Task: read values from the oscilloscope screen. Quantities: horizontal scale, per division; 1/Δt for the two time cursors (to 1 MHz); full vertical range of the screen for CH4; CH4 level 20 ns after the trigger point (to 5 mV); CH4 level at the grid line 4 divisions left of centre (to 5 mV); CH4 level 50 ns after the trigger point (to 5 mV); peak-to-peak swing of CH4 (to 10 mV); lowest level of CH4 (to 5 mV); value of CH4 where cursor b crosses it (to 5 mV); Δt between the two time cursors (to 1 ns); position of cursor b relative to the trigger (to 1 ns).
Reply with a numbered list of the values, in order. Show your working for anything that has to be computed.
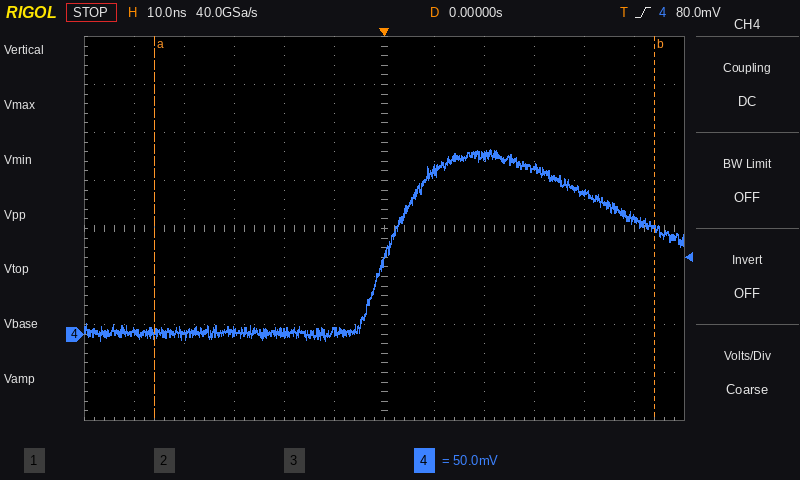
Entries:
1. 10 ns
2. 1 / 100 ns ≈ 10 MHz
3. 400 mV
4. 185 mV
5. 0 mV
6. 120 mV
7. 200 mV
8. -5 mV
9. 110 mV
10. 100 ns
11. +54 ns
